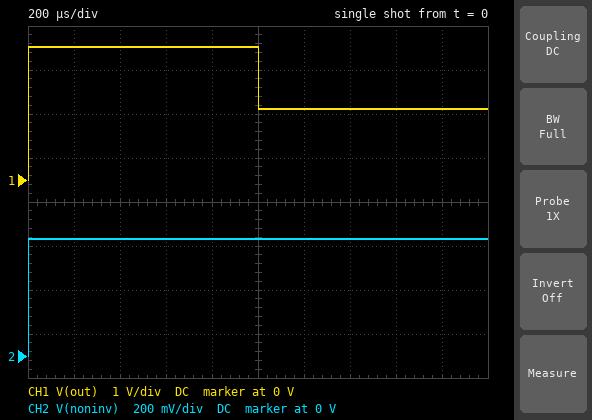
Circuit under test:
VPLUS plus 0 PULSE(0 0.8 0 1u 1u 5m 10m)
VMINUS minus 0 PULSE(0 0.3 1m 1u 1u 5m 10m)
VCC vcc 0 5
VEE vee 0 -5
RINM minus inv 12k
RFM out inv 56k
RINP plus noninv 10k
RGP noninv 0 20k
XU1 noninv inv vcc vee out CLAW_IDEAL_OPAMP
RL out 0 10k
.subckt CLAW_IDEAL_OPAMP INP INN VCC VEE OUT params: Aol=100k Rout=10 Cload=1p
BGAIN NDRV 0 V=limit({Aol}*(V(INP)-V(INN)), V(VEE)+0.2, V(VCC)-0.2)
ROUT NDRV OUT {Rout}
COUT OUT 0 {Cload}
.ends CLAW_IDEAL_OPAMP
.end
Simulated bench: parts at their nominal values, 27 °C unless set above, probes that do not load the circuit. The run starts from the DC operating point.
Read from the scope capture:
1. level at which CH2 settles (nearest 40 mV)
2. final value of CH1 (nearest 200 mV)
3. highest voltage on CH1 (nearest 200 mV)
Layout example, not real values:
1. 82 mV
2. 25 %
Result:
1. 520 mV
2. 1.6 V
3. 3.0 V
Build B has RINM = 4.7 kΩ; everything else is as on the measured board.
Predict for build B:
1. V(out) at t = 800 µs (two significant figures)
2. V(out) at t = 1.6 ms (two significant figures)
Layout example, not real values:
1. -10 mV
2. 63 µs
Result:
1. 4.8 V
2. 3.3 V
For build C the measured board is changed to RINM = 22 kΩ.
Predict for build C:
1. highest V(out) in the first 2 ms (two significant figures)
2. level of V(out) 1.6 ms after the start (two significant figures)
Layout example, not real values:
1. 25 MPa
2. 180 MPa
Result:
1. 1.9 V
2. 1.1 V
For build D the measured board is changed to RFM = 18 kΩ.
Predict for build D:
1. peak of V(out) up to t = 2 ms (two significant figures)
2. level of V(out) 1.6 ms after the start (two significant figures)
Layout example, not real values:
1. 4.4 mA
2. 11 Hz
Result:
1. 1.3 V
2. 880 mV
